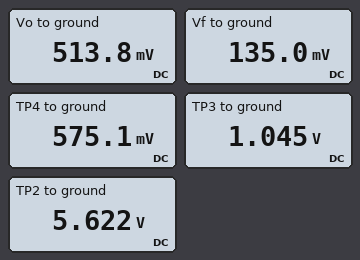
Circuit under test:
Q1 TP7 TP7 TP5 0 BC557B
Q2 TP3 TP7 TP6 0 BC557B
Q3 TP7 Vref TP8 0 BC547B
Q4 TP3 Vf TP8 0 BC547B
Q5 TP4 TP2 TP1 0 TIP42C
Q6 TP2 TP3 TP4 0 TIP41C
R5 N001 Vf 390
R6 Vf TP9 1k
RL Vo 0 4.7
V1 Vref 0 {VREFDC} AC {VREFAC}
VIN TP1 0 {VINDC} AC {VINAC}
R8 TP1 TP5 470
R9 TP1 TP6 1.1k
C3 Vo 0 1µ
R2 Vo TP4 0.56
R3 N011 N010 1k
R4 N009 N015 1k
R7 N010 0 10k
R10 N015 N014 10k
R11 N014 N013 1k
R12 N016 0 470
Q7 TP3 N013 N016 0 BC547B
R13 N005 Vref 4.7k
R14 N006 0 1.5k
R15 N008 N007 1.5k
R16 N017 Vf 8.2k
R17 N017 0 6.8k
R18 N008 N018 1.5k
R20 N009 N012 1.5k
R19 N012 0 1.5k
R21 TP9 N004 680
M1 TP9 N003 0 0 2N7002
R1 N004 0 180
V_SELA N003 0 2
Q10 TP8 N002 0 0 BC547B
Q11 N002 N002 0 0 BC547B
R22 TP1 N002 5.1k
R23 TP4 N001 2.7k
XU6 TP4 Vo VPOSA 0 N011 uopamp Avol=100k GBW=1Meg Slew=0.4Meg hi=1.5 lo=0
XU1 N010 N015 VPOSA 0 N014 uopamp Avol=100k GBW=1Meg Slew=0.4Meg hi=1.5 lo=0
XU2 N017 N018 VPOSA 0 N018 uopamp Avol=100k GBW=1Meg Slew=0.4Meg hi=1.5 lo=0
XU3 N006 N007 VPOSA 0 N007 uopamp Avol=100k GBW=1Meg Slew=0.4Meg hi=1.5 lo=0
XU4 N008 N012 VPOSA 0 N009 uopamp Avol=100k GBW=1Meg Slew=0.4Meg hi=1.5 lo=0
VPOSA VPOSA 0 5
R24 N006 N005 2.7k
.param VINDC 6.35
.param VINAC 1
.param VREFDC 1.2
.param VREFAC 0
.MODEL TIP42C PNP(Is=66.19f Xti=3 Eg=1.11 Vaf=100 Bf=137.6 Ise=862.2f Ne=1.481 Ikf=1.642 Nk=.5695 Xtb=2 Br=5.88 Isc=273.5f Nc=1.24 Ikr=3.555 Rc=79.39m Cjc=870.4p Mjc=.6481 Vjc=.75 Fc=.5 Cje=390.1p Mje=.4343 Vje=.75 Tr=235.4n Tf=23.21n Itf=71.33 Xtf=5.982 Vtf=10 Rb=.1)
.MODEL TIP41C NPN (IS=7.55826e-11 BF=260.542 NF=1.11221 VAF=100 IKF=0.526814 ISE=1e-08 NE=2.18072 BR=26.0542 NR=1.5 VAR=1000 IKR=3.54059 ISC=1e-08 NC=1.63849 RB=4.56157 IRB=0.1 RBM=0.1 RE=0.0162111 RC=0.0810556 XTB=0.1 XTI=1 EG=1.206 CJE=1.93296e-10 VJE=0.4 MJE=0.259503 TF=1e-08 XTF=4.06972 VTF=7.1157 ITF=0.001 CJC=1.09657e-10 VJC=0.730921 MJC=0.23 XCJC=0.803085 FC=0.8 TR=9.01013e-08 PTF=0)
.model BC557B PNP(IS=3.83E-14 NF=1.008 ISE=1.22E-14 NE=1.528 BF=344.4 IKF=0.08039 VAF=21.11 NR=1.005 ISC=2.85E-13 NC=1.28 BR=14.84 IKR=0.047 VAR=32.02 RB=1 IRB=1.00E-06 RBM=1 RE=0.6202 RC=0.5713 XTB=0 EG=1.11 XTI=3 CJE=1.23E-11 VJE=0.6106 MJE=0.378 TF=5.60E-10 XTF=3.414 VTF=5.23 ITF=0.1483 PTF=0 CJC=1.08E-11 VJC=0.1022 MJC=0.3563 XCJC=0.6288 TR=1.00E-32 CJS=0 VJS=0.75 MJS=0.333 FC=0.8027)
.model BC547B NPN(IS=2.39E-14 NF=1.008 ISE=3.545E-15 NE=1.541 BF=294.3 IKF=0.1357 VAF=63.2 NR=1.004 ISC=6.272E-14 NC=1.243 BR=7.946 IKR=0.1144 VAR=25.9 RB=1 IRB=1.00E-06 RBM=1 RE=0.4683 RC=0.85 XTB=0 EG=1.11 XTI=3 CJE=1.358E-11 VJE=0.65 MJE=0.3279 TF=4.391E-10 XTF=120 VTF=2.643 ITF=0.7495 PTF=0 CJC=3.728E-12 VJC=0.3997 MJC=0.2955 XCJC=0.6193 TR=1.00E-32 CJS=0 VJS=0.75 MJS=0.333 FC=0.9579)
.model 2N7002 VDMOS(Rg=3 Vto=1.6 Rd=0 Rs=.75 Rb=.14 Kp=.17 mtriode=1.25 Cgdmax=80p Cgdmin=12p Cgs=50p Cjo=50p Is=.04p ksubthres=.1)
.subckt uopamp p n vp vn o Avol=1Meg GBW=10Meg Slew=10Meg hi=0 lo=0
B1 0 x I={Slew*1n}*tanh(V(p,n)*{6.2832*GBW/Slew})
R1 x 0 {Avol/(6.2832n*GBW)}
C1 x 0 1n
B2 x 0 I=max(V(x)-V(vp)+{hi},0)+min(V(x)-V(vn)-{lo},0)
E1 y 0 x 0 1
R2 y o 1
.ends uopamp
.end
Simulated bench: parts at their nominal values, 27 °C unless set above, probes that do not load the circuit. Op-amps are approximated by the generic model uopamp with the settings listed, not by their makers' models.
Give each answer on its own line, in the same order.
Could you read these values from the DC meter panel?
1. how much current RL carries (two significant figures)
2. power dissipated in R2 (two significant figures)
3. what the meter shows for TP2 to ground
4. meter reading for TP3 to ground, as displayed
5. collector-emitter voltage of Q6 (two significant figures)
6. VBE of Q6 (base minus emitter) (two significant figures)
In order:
110 mA
6.7 mW
5.622 V
1.045 V
5.0 V
470 mV
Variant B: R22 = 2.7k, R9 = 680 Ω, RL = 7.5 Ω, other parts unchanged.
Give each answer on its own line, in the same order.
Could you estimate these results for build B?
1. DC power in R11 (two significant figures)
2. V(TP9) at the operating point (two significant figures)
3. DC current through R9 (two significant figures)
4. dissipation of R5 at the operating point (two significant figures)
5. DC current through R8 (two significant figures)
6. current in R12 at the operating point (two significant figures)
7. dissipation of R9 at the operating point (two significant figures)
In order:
2.1 mW
2.5 mV
1.5 mA
19 µW
2.1 mA
2.9 mA
1.4 mW
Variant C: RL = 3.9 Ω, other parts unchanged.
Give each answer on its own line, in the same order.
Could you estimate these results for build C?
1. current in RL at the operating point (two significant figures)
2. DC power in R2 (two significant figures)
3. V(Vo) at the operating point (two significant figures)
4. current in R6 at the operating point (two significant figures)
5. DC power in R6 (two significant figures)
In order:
130 mA
9.1 mW
500 mV
130 µA
17 µW
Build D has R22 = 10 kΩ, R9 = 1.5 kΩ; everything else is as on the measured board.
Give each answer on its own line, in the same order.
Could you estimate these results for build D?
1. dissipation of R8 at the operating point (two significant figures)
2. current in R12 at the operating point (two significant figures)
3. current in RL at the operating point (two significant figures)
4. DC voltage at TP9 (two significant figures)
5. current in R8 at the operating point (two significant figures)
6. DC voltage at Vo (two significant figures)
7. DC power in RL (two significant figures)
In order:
150 µW
2.0 mA
92 mA
1.4 mV
570 µA
430 mV
40 mW
